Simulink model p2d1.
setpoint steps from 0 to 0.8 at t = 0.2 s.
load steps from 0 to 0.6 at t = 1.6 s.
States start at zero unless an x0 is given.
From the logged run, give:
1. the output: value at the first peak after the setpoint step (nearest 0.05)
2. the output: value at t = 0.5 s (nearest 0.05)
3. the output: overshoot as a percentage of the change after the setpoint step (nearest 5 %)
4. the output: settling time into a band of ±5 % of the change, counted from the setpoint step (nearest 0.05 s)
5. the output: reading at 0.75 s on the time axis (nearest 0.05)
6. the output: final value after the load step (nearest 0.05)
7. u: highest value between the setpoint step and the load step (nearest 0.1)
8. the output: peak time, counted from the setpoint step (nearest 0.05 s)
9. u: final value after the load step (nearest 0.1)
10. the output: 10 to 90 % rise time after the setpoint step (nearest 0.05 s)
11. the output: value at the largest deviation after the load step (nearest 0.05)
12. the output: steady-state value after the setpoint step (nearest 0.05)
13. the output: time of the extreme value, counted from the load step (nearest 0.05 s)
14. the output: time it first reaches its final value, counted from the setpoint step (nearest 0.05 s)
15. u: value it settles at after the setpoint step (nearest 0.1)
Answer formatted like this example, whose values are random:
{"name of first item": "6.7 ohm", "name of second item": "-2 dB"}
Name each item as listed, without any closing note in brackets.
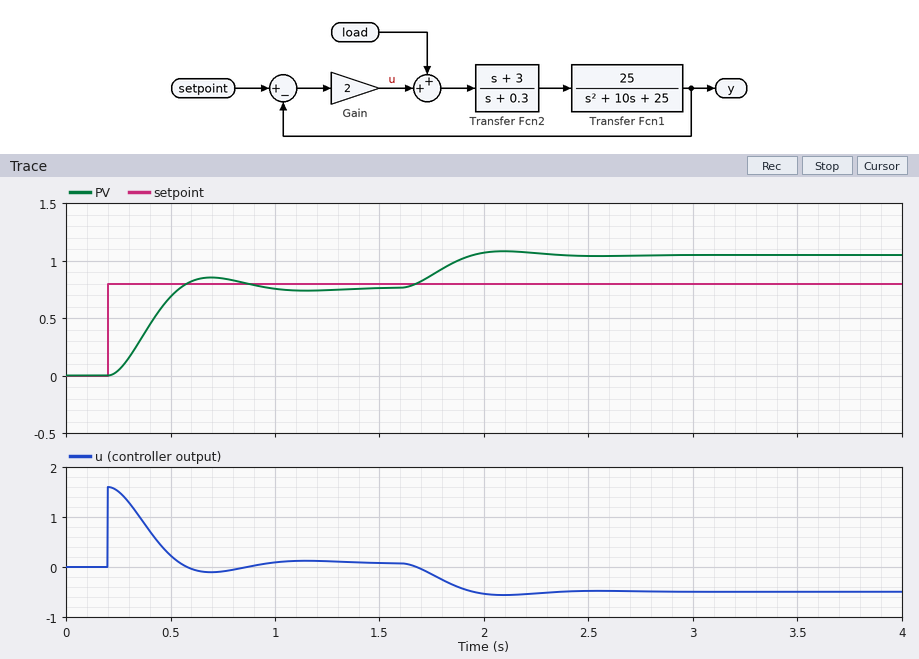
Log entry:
{"the output: value at the first peak after the setpoint step": "0.85", "the output: value at t = 0.5 s": "0.70", "the output: overshoot as a percentage of the change after the setpoint step": "10 %", "the output: settling time into a band of ±5 % of the change, counted from the setpoint step": "0.65 s", "the output: reading at 0.75 s on the time axis": "0.85", "the output: final value after the load step": "1.05", "u: highest value between the setpoint step and the load step": "1.6", "the output: peak time, counted from the setpoint step": "0.50 s", "u: final value after the load step": "-0.5", "the output: 10 to 90 % rise time after the setpoint step": "0.25 s", "the output: value at the largest deviation after the load step": "1.10", "the output: steady-state value after the setpoint step": "0.75", "the output: time of the extreme value, counted from the load step": "0.50 s", "the output: time it first reaches its final value, counted from the setpoint step": "0.35 s", "u: value it settles at after the setpoint step": "0.1"}
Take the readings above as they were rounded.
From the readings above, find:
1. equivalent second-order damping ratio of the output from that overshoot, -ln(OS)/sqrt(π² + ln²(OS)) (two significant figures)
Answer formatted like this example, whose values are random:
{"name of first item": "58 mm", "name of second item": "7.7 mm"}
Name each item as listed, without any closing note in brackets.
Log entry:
{"equivalent second-order damping ratio of the output from that overshoot, -ln(OS)/sqrt(π² + ln²(OS))": "0.59"}
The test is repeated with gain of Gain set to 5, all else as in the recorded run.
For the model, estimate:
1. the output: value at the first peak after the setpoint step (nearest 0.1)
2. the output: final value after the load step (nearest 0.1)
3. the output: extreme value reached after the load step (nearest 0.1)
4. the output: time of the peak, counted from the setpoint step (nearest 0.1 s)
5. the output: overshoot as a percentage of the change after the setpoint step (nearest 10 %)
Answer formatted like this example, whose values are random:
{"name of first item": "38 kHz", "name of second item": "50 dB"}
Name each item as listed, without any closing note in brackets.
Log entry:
{"the output: value at the first peak after the setpoint step": "1.0", "the output: final value after the load step": "0.9", "the output: extreme value reached after the load step": "0.9", "the output: time of the peak, counted from the setpoint step": "0.3 s", "the output: overshoot as a percentage of the change after the setpoint step": "30 %"}
